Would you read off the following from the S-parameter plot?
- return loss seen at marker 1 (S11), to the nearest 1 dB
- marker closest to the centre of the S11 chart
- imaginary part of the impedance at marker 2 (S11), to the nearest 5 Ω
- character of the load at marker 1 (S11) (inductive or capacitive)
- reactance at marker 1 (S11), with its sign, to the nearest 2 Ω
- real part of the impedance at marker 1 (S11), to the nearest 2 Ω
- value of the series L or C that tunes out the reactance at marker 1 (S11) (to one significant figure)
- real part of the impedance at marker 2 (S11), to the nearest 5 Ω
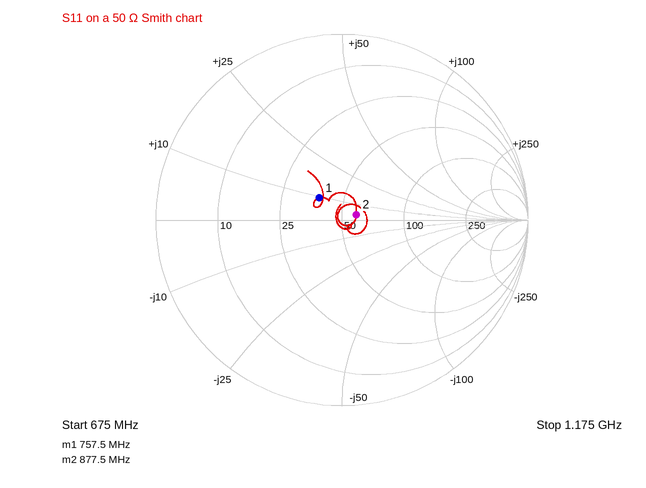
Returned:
15 dB
marker 2
+5 Ω
inductive
+10 Ω
38 Ω
20 pF
60 Ω
